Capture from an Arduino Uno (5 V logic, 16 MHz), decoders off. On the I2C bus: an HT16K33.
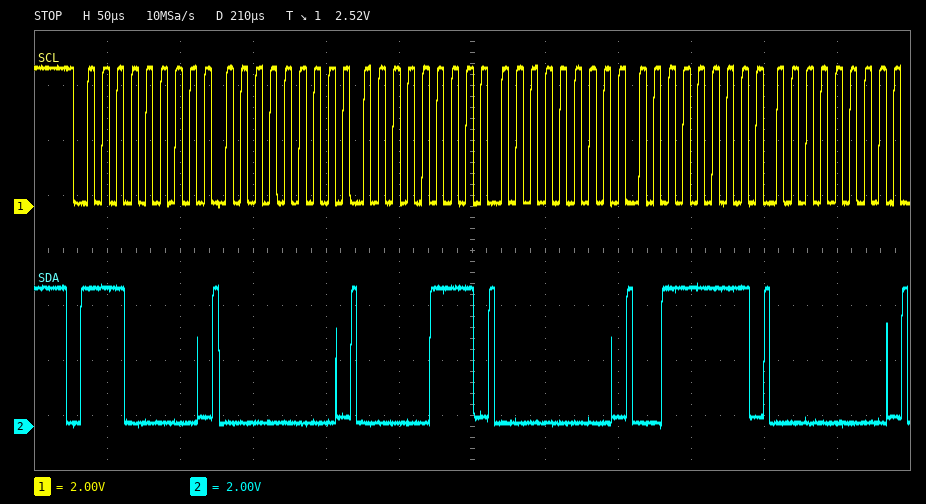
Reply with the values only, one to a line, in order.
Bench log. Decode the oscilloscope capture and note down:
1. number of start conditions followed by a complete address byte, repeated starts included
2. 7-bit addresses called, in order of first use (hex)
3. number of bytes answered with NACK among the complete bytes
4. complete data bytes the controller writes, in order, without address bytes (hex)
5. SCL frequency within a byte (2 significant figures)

1
0x70
0
00 07 00 3F 00
100 kHz
